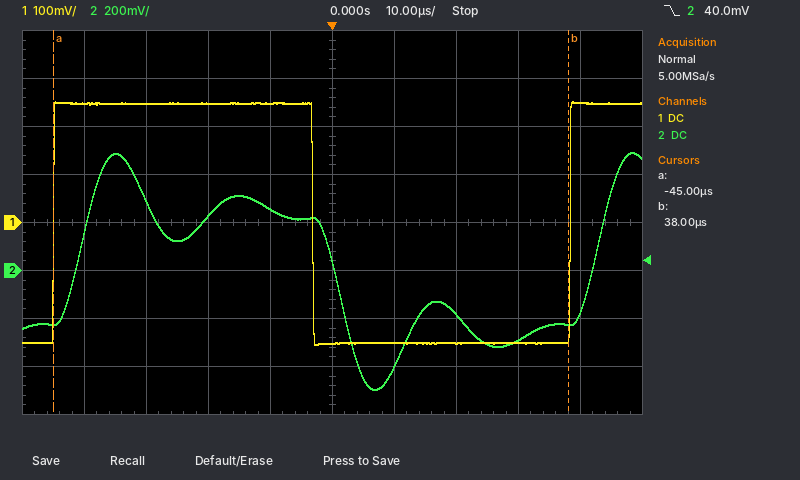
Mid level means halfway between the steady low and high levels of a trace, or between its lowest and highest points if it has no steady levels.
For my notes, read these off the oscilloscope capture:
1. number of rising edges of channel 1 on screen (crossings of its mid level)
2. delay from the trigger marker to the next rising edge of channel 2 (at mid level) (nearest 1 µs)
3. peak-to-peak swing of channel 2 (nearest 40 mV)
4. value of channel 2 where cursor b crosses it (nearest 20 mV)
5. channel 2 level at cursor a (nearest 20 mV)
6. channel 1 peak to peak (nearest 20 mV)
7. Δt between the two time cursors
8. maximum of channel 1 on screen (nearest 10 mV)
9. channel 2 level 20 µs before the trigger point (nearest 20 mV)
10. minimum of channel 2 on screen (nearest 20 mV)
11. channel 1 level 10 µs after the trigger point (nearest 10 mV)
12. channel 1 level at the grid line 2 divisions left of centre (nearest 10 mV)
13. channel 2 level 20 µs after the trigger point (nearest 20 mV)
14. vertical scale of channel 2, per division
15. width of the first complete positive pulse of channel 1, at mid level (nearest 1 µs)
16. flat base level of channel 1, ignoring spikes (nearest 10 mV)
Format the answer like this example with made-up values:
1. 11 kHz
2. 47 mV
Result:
1. 2
2. 42 µs
3. 1.00 V
4. -220 mV
5. -220 mV
6. 500 mV
7. 83 µs
8. 250 mV
9. 220 mV
10. -500 mV
11. -250 mV
12. 250 mV
13. -180 mV
14. 200 mV
15. 42 µs
16. -250 mV
